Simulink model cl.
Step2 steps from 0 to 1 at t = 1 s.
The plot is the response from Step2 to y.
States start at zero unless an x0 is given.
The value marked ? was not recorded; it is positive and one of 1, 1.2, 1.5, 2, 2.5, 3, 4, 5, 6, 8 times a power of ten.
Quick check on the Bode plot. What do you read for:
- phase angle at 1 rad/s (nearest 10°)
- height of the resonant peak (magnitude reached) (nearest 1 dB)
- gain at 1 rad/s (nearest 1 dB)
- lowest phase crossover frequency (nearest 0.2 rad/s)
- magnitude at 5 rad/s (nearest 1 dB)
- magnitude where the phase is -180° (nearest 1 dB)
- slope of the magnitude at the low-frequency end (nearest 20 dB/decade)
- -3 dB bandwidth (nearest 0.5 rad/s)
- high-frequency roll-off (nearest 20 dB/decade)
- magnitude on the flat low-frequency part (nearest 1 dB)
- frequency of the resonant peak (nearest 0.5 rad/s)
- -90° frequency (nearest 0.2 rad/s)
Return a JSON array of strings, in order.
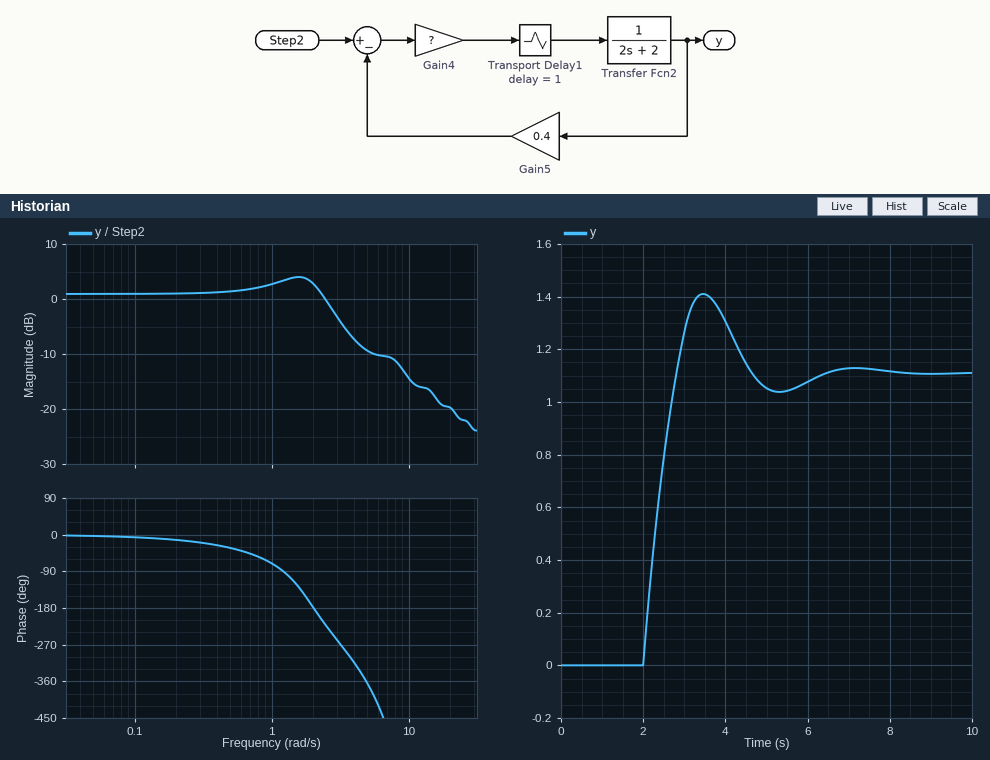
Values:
["-70°", "4 dB", "3 dB", "2.0 rad/s", "-9 dB", "3 dB", "0 dB/decade", "3.0 rad/s", "-20 dB/decade", "1 dB", "1.5 rad/s", "1.2 rad/s"]
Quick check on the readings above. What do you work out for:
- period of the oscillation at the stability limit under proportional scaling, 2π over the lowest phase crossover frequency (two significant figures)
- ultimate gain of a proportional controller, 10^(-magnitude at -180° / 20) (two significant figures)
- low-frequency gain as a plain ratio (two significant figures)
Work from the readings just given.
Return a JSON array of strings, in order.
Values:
["3.1 s", "0.71", "1.1"]
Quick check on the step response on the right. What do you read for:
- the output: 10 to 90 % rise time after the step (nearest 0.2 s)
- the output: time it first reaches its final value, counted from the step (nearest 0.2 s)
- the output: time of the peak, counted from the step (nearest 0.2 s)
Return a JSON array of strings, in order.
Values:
["0.6 s", "1.8 s", "2.4 s"]
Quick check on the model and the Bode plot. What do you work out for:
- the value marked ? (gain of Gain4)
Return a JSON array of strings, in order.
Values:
["4"]
